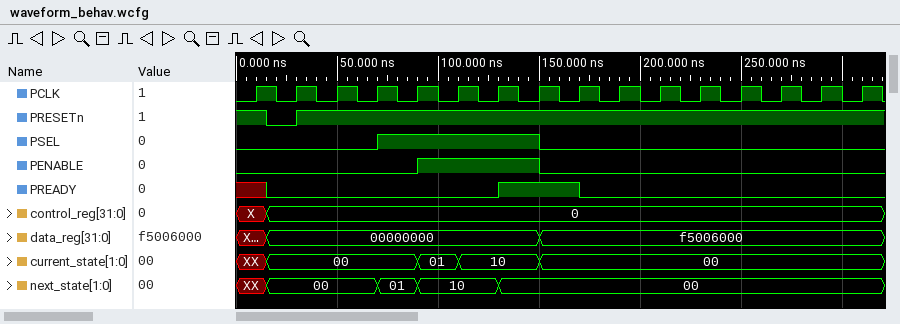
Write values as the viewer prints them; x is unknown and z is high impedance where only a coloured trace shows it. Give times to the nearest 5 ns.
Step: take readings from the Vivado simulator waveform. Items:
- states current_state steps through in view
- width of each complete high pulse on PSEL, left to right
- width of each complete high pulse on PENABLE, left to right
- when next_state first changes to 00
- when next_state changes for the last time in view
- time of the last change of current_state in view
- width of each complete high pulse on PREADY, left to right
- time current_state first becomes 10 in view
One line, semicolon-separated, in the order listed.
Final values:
XX, 00, 01, 10, 00; 80 ns; 60 ns; 15 ns; 130 ns; 150 ns; 40 ns; 110 ns
